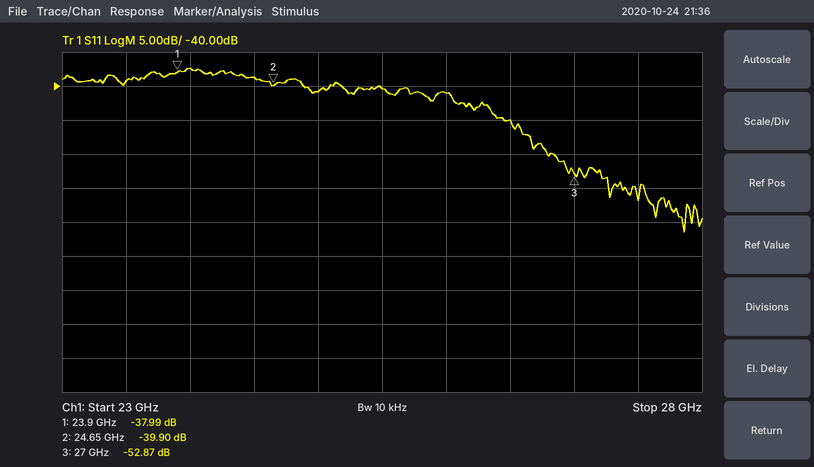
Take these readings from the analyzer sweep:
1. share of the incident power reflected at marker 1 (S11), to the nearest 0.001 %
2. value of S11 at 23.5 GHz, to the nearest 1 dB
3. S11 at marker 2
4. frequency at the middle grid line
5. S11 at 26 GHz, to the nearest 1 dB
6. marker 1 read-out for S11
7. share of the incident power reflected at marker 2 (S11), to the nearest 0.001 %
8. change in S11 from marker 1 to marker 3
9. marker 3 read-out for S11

0.016 %
-39 dB
-39.90 dB
25.5 GHz
-41 dB
-37.99 dB
0.010 %
-14.88 dB
-52.87 dB
